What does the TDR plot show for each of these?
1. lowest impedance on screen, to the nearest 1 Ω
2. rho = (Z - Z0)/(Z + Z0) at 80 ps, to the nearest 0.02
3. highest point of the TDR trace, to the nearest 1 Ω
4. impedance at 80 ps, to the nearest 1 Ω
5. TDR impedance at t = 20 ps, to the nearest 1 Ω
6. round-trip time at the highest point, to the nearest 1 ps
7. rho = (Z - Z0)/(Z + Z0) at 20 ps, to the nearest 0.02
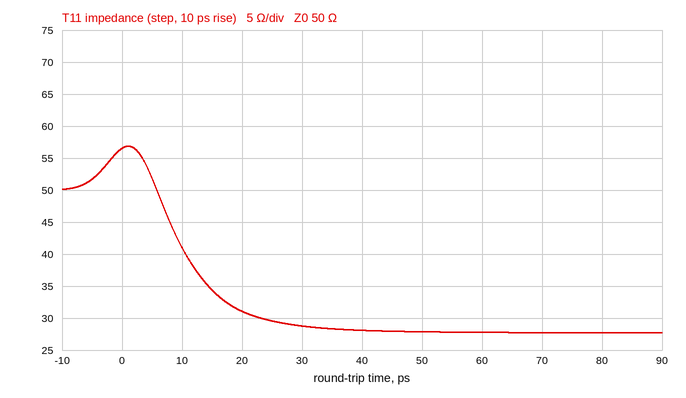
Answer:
28 Ω
-0.28
57 Ω
28 Ω
31 Ω
1 ps
-0.24
